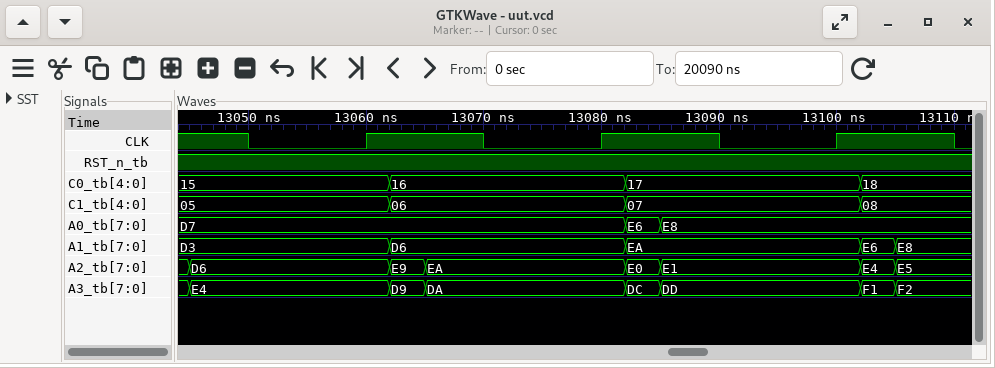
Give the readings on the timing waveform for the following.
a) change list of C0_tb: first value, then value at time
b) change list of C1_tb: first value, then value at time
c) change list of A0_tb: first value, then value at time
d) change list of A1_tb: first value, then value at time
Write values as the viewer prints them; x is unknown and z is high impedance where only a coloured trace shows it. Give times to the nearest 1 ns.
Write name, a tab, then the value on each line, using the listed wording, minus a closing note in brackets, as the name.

change list of C0_tb: first value, then value at time	15, 16 at 13062 ns, 17 at 13082 ns, 18 at 13102 ns
change list of C1_tb: first value, then value at time	05, 06 at 13062 ns, 07 at 13082 ns, 08 at 13102 ns
change list of A0_tb: first value, then value at time	D7, E6 at 13082 ns, E8 at 13085 ns
change list of A1_tb: first value, then value at time	D3, D6 at 13062 ns, EA at 13082 ns, E6 at 13102 ns, E8 at 13105 ns
